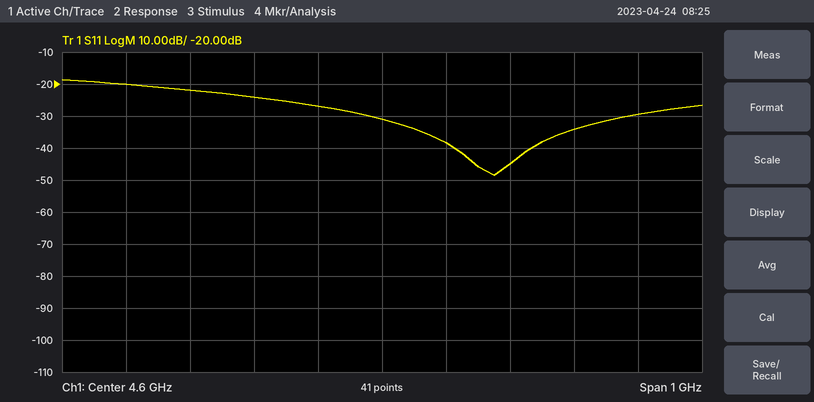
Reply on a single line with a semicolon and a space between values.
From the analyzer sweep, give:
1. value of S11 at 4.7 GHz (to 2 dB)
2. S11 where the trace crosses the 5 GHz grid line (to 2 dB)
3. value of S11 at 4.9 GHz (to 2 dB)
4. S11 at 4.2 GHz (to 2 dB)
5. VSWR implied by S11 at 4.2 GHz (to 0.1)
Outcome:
-38 dB; -30 dB; -34 dB; -20 dB; 1.2
